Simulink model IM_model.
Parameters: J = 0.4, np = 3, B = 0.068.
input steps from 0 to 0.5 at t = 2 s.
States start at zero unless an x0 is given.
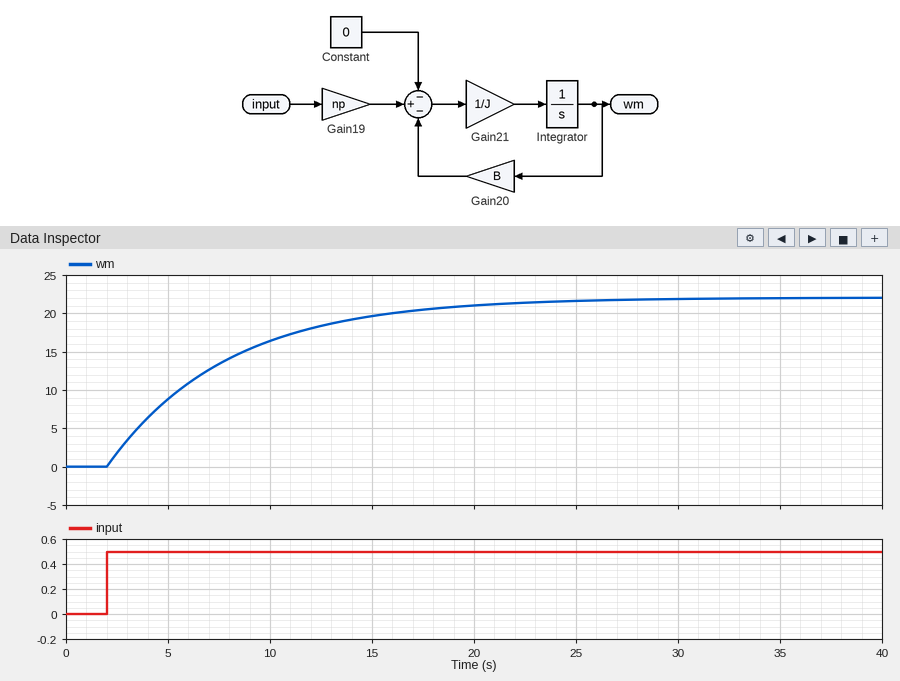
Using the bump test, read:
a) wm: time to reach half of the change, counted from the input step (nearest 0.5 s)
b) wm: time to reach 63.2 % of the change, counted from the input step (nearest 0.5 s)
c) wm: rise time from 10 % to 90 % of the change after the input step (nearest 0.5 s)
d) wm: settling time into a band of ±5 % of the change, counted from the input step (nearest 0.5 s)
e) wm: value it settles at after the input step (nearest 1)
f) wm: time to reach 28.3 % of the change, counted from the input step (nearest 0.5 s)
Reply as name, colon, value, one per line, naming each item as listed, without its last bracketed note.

wm: time to reach half of the change, counted from the input step: 4.0 s
wm: time to reach 63.2 % of the change, counted from the input step: 6.0 s
wm: rise time from 10 % to 90 % of the change after the input step: 13.0 s
wm: settling time into a band of ±5 % of the change, counted from the input step: 17.5 s
wm: value it settles at after the input step: 22
wm: time to reach 28.3 % of the change, counted from the input step: 2.0 s
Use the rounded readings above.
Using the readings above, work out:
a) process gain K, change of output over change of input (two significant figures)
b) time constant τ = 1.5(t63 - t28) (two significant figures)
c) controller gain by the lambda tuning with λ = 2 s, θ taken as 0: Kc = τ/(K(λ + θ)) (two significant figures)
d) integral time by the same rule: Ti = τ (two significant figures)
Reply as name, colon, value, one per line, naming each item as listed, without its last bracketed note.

process gain K, change of output over change of input: 44
time constant τ = 1.5(t63 - t28): 6.0 s
controller gain by the lambda tuning with λ = 2 s, θ taken as 0: Kc = τ/(K(λ + θ)): 0.068
integral time by the same rule: Ti = τ: 6.0 s
